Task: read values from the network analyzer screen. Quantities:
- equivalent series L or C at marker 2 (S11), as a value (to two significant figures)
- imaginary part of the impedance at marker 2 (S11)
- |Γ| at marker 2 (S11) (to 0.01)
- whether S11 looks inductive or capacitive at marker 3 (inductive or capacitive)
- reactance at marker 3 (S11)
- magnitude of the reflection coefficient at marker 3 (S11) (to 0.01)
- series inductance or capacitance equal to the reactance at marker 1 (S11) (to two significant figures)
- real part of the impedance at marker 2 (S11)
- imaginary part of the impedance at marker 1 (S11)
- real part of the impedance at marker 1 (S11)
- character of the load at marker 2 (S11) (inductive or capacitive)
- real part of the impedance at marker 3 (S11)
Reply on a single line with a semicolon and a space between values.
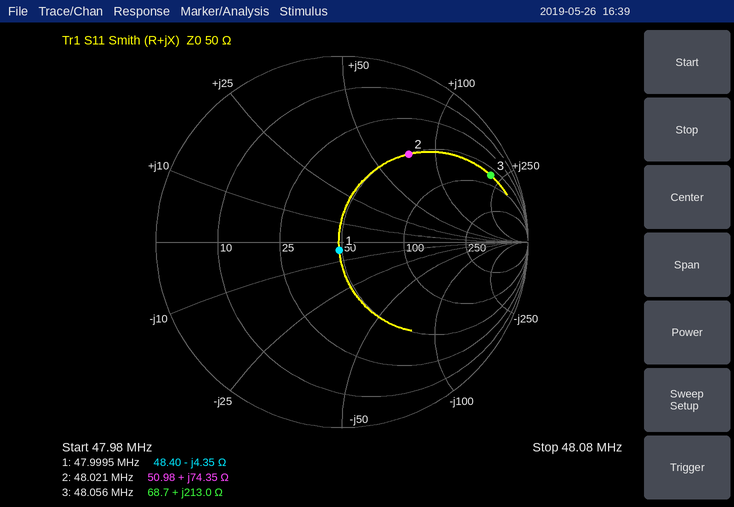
250 nH; +74.35 Ω; 0.59; inductive; +213.0 Ω; 0.88; 760 pF; 50.98 Ω; -4.35 Ω; 48.40 Ω; inductive; 68.7 Ω
